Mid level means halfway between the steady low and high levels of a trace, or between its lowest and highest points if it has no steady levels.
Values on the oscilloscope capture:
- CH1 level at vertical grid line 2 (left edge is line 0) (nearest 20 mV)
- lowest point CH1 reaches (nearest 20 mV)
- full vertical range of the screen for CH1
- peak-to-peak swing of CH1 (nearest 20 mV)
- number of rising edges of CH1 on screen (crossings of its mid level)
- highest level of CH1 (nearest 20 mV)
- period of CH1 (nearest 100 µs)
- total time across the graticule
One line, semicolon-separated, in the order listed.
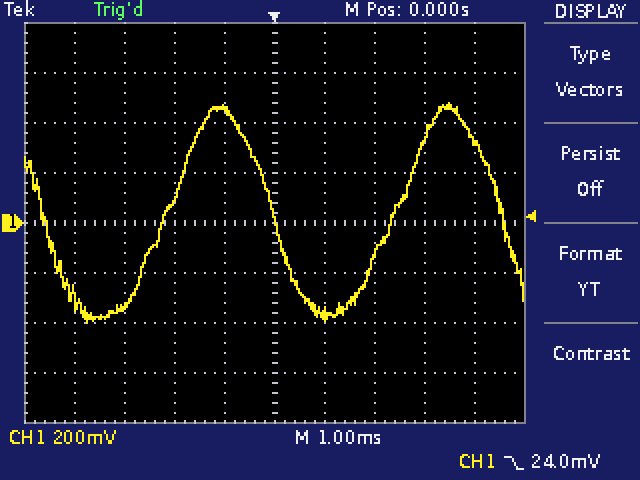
-340 mV; -400 mV; 1.6 V; 880 mV; 2; 480 mV; 4.6 ms; 10 ms
